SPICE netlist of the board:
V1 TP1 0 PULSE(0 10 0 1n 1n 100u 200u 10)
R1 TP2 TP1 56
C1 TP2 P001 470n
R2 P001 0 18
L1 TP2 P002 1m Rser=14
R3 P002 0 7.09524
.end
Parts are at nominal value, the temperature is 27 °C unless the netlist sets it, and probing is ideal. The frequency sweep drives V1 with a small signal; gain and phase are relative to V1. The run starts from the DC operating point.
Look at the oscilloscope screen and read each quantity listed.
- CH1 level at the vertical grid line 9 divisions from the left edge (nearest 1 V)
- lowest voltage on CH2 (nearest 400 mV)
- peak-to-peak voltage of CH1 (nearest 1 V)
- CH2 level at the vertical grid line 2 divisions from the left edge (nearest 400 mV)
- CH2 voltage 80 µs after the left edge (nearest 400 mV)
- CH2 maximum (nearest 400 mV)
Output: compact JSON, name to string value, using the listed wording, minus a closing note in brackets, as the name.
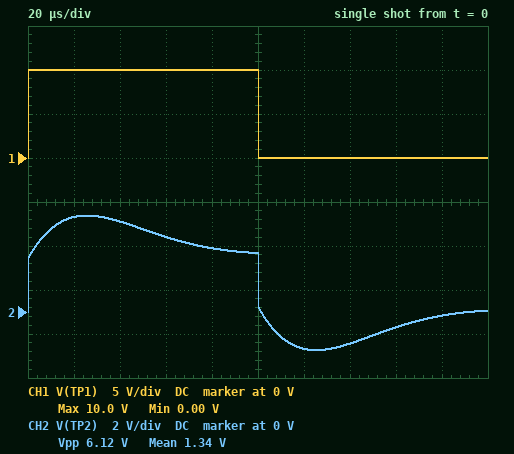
{"CH1 level at the vertical grid line 9 divisions from the left edge": "0 V", "lowest voltage on CH2": "-1.6 V", "peak-to-peak voltage of CH1": "10 V", "CH2 level at the vertical grid line 2 divisions from the left edge": "4.0 V", "CH2 voltage 80 µs after the left edge": "2.8 V", "CH2 maximum": "4.4 V"}
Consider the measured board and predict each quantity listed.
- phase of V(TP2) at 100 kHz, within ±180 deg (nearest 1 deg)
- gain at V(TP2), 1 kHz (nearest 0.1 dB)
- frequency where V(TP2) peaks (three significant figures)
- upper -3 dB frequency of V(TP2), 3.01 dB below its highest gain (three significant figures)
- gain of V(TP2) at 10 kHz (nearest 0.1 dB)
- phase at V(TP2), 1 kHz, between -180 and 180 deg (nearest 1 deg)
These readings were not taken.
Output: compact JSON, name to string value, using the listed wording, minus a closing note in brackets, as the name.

{"phase of V(TP2) at 100 kHz, within ±180 deg": "-7 deg", "gain at V(TP2), 1 kHz": "-10.9 dB", "frequency where V(TP2) peaks": "7.36 kHz", "upper -3 dB frequency of V(TP2), 3.01 dB below its highest gain": "16.3 kHz", "gain of V(TP2) at 10 kHz": "-6.1 dB", "phase at V(TP2), 1 kHz, between -180 and 180 deg": "9 deg"}
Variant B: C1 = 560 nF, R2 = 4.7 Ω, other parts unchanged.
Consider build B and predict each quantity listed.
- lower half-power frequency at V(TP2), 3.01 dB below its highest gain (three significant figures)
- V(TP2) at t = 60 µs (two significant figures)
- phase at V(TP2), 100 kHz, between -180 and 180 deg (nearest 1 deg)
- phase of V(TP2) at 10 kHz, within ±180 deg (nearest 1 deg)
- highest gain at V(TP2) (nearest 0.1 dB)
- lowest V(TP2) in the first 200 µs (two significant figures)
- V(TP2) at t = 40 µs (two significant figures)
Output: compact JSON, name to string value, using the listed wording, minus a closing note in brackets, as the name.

{"lower half-power frequency at V(TP2), 3.01 dB below its highest gain": "3.54 kHz", "V(TP2) at t = 60 µs": "3.8 V", "phase at V(TP2), 100 kHz, between -180 and 180 deg": "-28 deg", "phase of V(TP2) at 10 kHz, within ±180 deg": "-35 deg", "highest gain at V(TP2)": "-4.5 dB", "lowest V(TP2) in the first 200 µs": "-2.1 V", "V(TP2) at t = 40 µs": "4.6 V"}
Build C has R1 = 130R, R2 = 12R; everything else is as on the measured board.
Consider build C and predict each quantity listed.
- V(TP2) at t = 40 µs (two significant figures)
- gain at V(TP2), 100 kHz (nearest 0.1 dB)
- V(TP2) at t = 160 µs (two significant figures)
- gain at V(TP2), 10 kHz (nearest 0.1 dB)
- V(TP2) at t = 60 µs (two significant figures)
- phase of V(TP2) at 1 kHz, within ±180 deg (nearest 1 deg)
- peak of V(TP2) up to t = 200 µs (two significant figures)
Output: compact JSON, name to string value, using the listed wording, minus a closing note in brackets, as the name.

{"V(TP2) at t = 40 µs": "2.5 V", "gain at V(TP2), 100 kHz": "-21.1 dB", "V(TP2) at t = 160 µs": "-510 mV", "gain at V(TP2), 10 kHz": "-10.2 dB", "V(TP2) at t = 60 µs": "1.9 V", "phase of V(TP2) at 1 kHz, within ±180 deg": "11 deg", "peak of V(TP2) up to t = 200 µs": "2.6 V"}
